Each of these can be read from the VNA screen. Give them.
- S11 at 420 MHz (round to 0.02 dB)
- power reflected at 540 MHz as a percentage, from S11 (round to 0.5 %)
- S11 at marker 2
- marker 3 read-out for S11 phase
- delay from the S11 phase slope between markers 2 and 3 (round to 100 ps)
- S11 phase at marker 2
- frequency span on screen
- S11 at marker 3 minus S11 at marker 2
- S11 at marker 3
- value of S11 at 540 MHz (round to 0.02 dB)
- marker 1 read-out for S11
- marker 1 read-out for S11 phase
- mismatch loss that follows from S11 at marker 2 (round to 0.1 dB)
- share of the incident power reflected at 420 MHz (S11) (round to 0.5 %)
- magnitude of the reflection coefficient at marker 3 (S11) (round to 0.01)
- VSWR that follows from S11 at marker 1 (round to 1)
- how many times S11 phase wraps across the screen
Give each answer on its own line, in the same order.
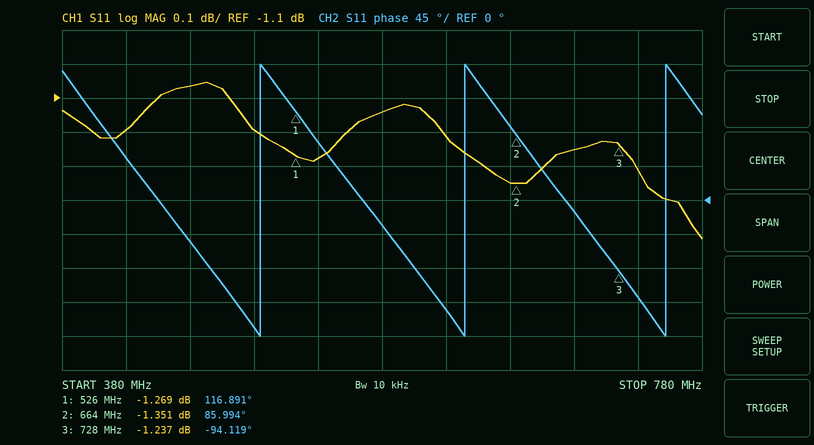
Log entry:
-1.20 dB
74.5 %
-1.351 dB
-94.119°
7.8 ns
85.994°
400 MHz
0.114 dB
-1.237 dB
-1.28 dB
-1.269 dB
116.891°
5.7 dB
76.0 %
0.87
14
3
